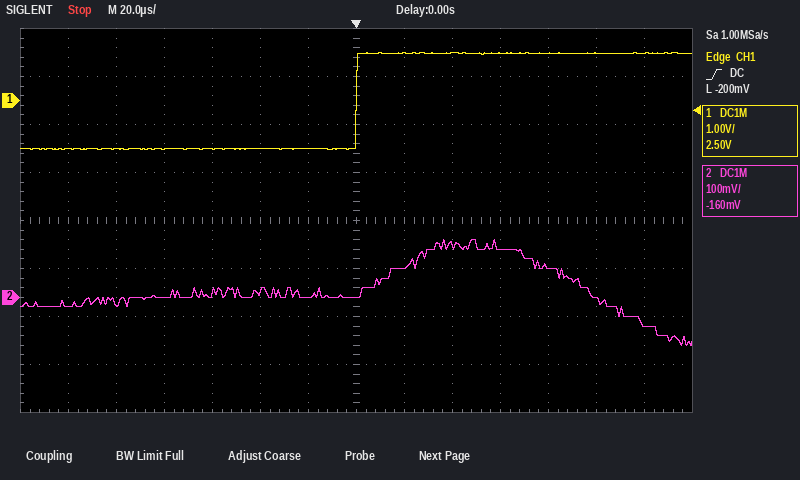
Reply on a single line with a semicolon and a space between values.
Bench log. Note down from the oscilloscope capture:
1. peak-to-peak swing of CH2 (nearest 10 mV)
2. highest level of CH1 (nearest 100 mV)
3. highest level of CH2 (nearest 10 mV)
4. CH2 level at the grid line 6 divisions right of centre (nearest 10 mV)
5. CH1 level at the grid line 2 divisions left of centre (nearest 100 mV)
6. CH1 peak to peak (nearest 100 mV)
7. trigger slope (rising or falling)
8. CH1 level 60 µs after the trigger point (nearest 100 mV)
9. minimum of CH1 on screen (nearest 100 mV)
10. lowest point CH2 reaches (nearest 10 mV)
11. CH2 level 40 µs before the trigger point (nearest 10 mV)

220 mV; 1.0 V; 120 mV; -60 mV; -1.0 V; 2.0 V; rising; 1.0 V; -1.0 V; -100 mV; 10 mV
